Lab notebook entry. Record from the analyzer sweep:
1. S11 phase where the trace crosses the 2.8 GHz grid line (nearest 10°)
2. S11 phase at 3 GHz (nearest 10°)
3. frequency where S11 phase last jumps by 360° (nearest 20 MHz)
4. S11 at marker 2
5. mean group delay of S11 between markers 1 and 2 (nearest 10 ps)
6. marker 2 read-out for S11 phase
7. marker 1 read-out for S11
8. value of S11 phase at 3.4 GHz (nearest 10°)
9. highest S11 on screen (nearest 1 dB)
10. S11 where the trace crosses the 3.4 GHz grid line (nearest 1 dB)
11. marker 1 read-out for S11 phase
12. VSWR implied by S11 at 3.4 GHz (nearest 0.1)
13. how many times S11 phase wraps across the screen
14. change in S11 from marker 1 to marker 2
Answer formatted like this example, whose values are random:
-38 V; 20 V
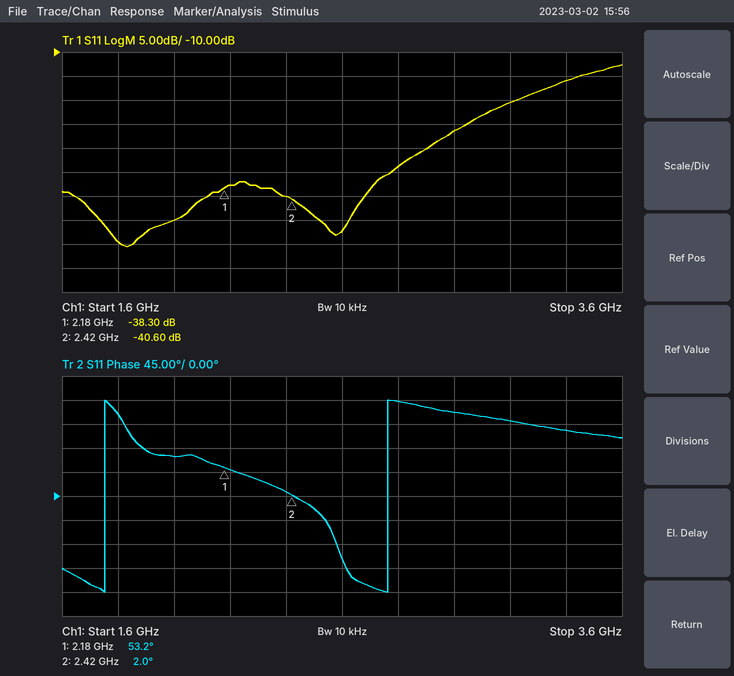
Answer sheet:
180°; 160°; 2.76 GHz; -40.60 dB; 590 ps; 2.0°; -38.30 dB; 120°; -13 dB; -16 dB; 53.2°; 1.4; 2; -2.30 dB
